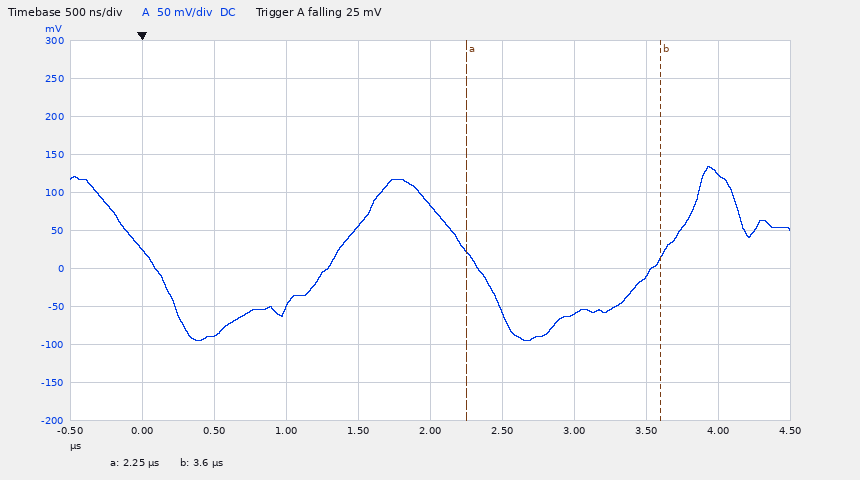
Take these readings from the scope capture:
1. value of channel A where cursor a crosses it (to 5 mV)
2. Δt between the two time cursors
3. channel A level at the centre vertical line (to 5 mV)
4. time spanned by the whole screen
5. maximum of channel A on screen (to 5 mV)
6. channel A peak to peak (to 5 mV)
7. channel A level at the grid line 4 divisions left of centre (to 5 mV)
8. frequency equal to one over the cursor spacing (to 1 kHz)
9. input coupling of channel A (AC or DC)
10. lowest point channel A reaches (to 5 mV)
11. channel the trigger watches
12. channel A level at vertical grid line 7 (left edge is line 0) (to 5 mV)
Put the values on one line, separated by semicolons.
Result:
20 mV; 1.35 µs; 85 mV; 5 µs; 135 mV; 230 mV; 25 mV; 741 kHz; DC; -95 mV; channel A; -60 mV
